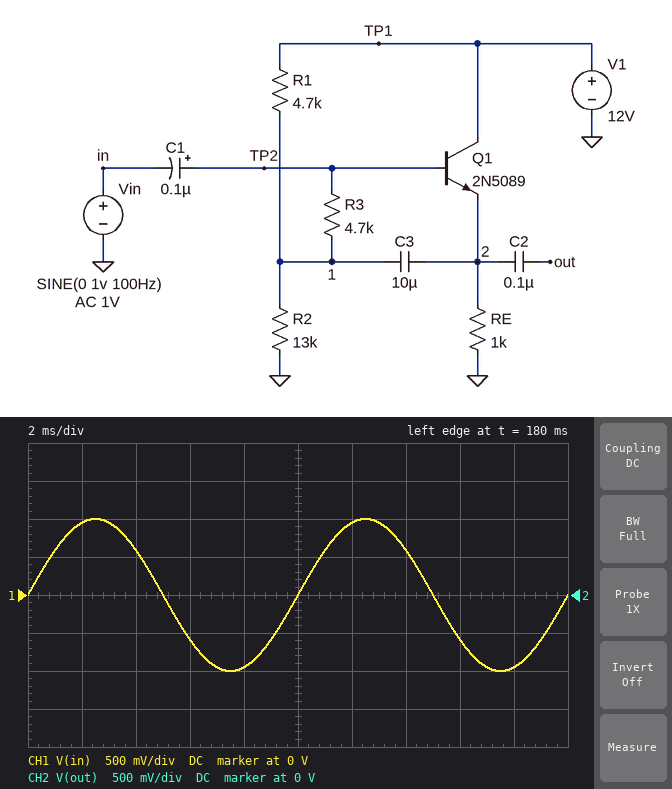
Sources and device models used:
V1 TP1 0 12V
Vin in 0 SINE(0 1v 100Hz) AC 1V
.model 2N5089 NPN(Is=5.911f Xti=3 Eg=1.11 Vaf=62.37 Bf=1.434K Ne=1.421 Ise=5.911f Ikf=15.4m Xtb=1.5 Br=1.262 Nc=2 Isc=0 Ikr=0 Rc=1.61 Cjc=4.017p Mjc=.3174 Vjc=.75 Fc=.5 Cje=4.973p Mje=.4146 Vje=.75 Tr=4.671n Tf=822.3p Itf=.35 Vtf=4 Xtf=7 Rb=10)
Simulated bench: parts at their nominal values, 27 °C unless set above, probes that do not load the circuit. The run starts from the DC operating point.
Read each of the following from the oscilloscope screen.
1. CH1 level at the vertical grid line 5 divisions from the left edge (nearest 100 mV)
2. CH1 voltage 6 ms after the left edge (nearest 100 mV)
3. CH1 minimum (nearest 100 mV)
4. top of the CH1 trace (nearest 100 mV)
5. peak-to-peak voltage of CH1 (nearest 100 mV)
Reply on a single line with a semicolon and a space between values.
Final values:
0 V; -600 mV; -1.0 V; 1.0 V; 2.0 V
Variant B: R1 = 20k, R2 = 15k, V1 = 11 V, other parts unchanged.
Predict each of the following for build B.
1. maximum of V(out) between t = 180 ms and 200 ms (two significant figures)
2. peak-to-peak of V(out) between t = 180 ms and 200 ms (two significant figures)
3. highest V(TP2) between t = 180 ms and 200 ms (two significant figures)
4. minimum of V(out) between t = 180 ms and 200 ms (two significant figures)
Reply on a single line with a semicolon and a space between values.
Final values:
5.0 V; 2.1 V; 5.7 V; 2.9 V
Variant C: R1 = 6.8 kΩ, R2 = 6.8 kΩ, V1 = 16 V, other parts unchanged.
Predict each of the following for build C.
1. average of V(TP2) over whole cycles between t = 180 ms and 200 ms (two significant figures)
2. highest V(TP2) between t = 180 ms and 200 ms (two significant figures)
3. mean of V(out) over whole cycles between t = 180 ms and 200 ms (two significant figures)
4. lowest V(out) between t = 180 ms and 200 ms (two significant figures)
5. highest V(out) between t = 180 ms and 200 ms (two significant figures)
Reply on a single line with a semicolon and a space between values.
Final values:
7.9 V; 9.1 V; 7.2 V; 6.0 V; 8.4 V
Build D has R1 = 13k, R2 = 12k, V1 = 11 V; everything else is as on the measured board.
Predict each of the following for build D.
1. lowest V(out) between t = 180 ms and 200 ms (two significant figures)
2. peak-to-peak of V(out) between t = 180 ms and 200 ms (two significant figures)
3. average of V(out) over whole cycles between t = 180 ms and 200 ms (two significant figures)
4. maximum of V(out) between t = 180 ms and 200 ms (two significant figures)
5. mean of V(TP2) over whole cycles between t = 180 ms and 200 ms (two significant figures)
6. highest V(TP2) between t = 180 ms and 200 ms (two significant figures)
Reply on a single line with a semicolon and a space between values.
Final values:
3.4 V; 2.2 V; 4.5 V; 5.6 V; 5.2 V; 6.3 V
